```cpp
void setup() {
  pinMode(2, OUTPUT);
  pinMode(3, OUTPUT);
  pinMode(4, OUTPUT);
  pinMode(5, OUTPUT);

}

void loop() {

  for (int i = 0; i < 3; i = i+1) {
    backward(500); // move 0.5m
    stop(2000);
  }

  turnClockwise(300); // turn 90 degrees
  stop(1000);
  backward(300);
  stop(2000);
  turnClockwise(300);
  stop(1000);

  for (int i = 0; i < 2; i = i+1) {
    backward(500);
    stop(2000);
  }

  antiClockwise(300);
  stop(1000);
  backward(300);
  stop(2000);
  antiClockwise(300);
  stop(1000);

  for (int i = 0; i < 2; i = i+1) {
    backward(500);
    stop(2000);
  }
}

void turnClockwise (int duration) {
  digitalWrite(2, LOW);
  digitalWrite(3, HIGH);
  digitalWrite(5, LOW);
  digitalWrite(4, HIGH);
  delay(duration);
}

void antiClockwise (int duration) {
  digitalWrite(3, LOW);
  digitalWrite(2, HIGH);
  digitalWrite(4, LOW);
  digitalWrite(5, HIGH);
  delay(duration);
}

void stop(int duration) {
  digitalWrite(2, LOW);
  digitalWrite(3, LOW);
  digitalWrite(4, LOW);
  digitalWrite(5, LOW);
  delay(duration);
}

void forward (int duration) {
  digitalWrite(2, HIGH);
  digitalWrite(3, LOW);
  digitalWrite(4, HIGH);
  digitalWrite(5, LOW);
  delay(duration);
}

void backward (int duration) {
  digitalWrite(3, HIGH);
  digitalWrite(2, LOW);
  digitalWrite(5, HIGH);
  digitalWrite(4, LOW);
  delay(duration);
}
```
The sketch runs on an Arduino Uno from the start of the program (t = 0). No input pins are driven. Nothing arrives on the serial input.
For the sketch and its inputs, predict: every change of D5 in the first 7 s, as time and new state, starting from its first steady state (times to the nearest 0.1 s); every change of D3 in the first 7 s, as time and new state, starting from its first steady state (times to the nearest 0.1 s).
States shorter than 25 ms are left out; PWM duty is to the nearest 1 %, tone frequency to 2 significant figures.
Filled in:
0 s high; 0.5 s low; 2.5 s high; 3 s low; 5 s high; 5.5 s low
0 s high; 0.5 s low; 2.5 s high; 3 s low; 5 s high; 5.5 s low
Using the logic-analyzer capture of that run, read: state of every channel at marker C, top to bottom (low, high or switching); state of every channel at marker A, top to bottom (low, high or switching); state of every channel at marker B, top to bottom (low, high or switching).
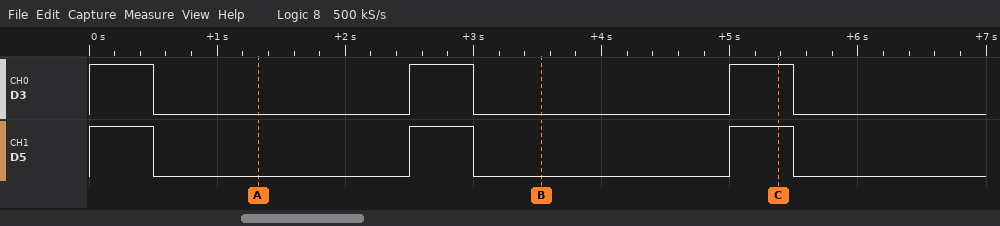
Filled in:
D3 high, D5 high
D3 low, D5 low
D3 low, D5 low
